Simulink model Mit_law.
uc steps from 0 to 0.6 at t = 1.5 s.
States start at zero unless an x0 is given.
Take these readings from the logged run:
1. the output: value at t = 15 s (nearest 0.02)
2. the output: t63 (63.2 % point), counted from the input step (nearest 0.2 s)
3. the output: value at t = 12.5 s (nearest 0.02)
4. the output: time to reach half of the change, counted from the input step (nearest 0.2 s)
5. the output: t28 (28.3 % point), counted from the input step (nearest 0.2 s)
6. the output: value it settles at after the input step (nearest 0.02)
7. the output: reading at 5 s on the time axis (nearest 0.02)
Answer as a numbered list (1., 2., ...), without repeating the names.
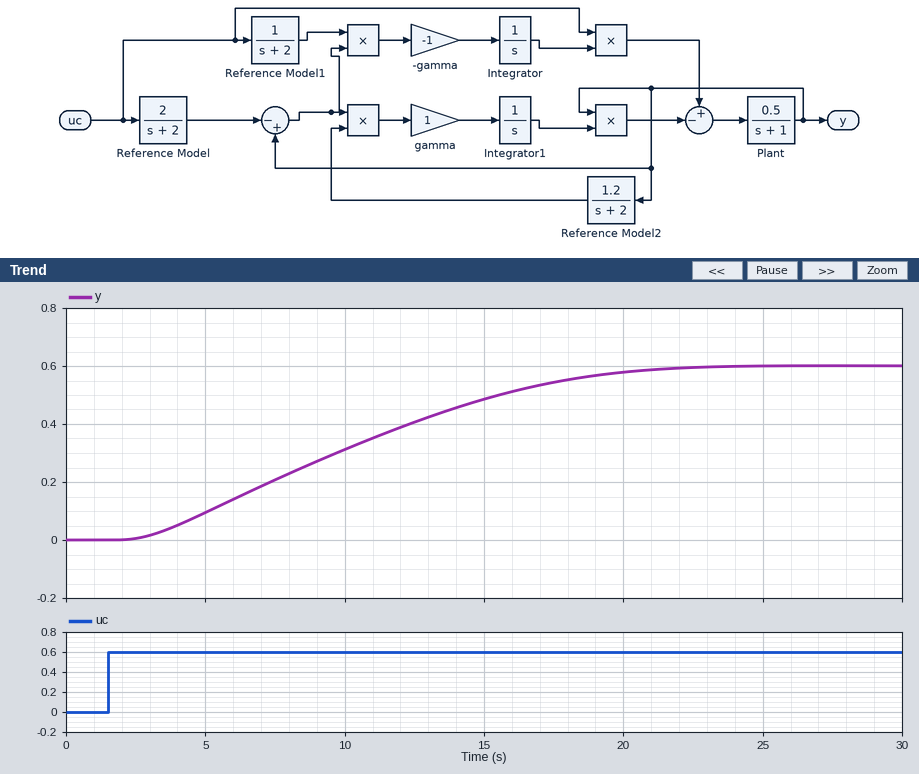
1. 0.48
2. 10.2 s
3. 0.40
4. 8.2 s
5. 5.2 s
6. 0.60
7. 0.10
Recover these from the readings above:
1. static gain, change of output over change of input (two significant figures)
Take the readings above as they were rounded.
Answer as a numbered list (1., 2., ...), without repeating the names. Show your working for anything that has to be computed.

1. (0.6 - 0) / (0.6 - 0) = 1.0
